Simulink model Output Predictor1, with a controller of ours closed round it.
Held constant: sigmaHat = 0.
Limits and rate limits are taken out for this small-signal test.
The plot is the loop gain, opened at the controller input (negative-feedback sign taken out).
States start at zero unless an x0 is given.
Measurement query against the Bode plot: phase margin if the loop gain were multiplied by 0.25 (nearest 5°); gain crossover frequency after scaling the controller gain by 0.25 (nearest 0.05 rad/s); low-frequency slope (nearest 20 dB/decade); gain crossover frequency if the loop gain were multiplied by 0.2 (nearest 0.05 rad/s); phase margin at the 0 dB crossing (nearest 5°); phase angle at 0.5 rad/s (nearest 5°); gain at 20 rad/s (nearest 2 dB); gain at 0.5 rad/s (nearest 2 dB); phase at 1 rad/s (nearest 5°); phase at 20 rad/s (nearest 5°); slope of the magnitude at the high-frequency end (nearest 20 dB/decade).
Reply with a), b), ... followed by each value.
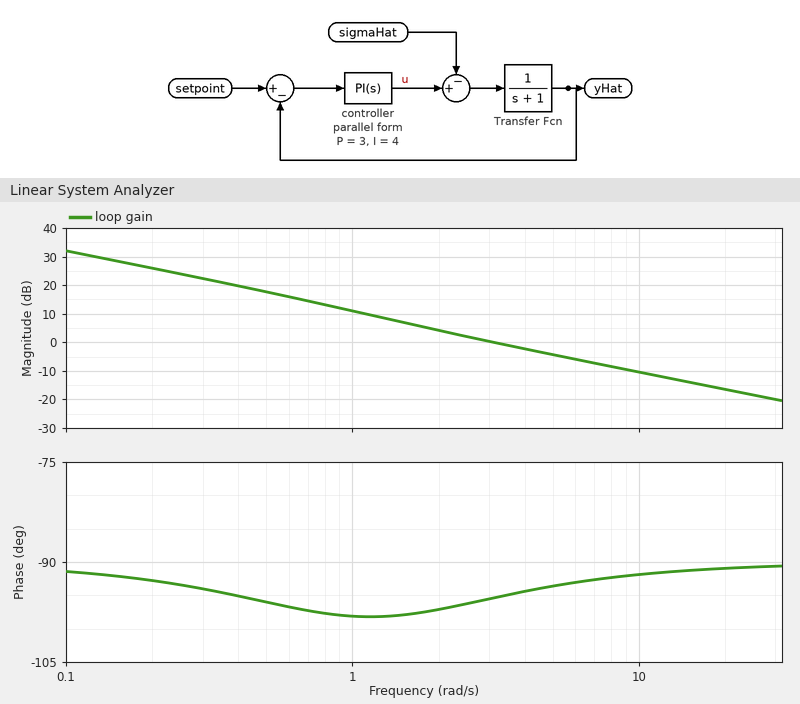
a) 80°
b) 0.90 rad/s
c) -20 dB/decade
d) 0.75 rad/s
e) 85°
f) -95°
g) -16 dB
h) 18 dB
i) -100°
j) -90°
k) -20 dB/decade
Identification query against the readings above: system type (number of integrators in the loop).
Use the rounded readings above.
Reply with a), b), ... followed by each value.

a) 1
